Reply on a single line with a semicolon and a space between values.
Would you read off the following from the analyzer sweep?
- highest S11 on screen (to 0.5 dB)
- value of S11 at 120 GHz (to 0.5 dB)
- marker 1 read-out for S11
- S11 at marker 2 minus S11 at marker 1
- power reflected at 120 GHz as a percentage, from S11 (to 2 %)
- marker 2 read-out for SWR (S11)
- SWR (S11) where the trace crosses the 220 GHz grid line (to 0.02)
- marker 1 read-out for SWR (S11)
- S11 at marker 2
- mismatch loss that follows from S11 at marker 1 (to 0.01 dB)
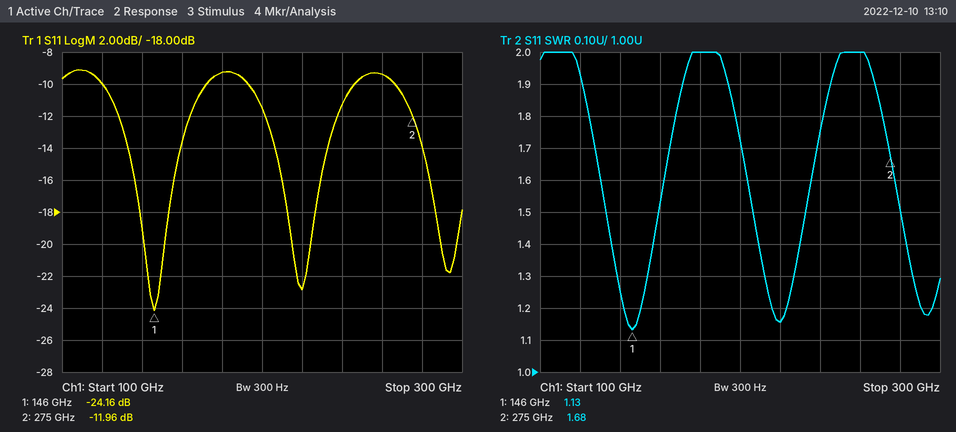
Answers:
-9.0 dB; -10.0 dB; -24.16 dB; 12.20 dB; 10 %; 1.68; 1.16; 1.13; -11.96 dB; 0.02 dB
